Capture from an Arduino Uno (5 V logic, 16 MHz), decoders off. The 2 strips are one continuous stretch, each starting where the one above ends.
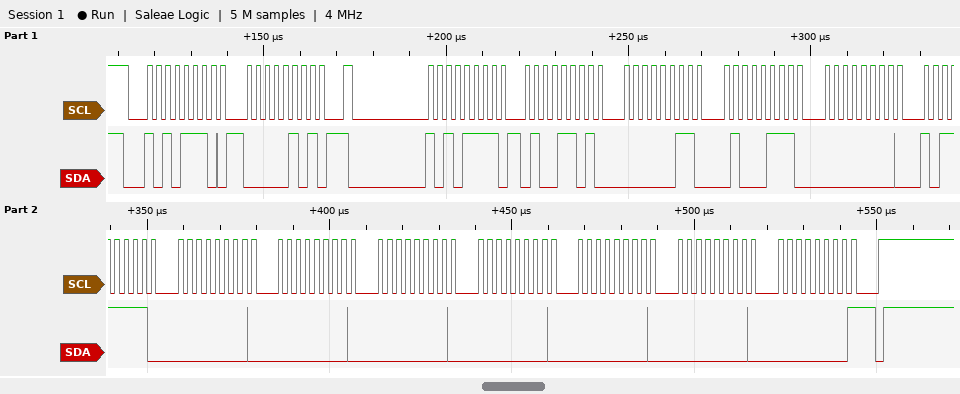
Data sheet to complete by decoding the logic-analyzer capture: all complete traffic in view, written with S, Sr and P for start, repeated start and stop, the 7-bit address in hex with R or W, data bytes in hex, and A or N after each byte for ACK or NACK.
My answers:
S 57W A 05 A Sr 57R A 4D A 03 A 47 A 00 A BF A 00 A 00 A 00 A 00 A 00 A 00 A 00 N P
